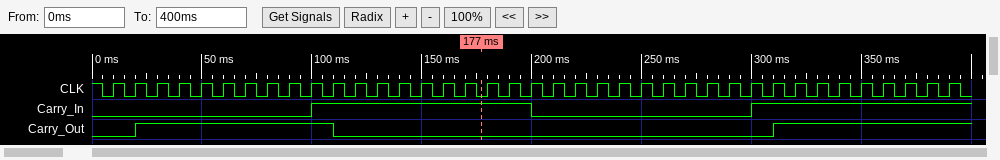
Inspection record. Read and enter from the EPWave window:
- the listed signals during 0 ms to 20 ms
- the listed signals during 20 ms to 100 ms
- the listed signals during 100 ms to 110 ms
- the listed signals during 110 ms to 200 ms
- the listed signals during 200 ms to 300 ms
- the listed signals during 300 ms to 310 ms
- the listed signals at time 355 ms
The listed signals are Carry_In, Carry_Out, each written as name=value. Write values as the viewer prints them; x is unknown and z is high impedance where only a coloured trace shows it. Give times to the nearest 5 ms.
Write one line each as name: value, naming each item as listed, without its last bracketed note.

the listed signals during 0 ms to 20 ms: Carry_In=0, Carry_Out=0
the listed signals during 20 ms to 100 ms: Carry_In=0, Carry_Out=1
the listed signals during 100 ms to 110 ms: Carry_In=1, Carry_Out=1
the listed signals during 110 ms to 200 ms: Carry_In=1, Carry_Out=0
the listed signals during 200 ms to 300 ms: Carry_In=0, Carry_Out=0
the listed signals during 300 ms to 310 ms: Carry_In=1, Carry_Out=0
the listed signals at time 355 ms: Carry_In=1, Carry_Out=1
